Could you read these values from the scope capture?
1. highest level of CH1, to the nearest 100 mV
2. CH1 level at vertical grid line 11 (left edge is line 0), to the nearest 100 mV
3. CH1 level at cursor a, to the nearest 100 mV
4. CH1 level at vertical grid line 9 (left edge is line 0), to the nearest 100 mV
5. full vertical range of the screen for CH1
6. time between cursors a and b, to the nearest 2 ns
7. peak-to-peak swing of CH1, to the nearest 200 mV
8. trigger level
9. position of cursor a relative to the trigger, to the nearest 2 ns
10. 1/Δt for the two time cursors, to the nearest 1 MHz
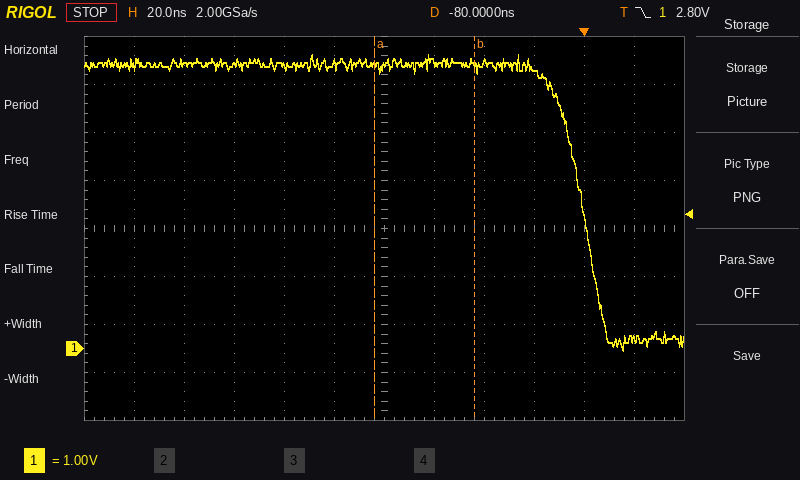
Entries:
6.1 V
200 mV
5.9 V
5.8 V
8 V
40 ns
6.2 V
2.80 V
-84 ns
25 MHz
